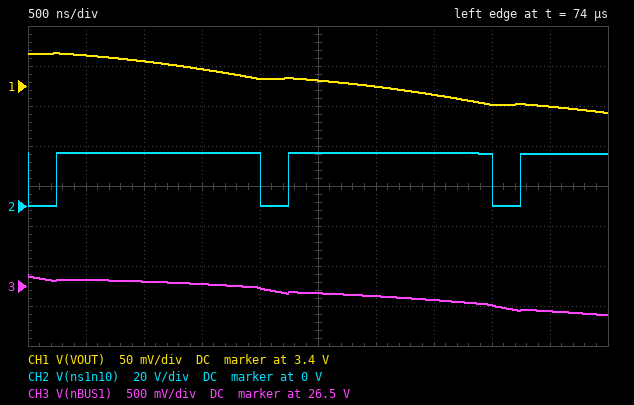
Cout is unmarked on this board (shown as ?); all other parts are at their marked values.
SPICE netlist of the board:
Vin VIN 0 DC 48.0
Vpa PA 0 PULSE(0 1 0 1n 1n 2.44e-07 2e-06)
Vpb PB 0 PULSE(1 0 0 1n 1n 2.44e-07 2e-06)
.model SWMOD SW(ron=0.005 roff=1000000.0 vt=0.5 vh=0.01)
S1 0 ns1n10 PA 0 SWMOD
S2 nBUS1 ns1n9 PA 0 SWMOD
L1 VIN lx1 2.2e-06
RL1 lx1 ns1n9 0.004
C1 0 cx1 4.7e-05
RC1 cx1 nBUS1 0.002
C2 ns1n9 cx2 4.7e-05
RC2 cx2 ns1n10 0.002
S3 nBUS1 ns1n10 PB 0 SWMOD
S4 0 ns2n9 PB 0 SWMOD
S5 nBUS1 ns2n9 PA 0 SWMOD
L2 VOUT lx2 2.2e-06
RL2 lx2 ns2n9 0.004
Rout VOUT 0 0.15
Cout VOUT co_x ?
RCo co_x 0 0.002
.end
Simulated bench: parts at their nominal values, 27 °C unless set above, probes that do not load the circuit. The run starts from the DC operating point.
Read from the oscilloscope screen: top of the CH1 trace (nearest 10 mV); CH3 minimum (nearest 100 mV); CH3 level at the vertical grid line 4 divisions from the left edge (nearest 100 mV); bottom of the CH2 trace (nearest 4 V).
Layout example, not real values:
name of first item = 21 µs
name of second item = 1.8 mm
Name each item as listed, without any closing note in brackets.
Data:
top of the CH1 trace = 3.44 V
CH3 minimum = 26.1 V
CH3 level at the vertical grid line 4 divisions from the left edge = 26.5 V
bottom of the CH2 trace = 0 V
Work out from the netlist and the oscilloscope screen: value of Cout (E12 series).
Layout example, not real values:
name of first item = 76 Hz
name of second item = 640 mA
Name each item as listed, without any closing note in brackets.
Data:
value of Cout = 150 µF
